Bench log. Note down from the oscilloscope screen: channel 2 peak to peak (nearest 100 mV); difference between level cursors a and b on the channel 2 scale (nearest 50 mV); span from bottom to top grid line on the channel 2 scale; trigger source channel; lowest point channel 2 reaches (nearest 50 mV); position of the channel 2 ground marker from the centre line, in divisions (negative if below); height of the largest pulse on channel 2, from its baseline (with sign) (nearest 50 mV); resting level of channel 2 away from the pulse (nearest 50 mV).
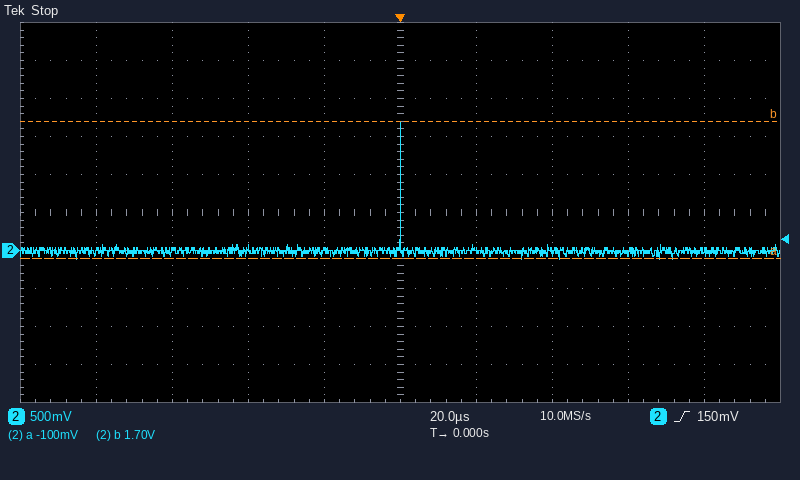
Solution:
1.80 V
1.80 V
5 V
channel 2
-100 mV
-1.0 div
+1.70 V
0 mV
